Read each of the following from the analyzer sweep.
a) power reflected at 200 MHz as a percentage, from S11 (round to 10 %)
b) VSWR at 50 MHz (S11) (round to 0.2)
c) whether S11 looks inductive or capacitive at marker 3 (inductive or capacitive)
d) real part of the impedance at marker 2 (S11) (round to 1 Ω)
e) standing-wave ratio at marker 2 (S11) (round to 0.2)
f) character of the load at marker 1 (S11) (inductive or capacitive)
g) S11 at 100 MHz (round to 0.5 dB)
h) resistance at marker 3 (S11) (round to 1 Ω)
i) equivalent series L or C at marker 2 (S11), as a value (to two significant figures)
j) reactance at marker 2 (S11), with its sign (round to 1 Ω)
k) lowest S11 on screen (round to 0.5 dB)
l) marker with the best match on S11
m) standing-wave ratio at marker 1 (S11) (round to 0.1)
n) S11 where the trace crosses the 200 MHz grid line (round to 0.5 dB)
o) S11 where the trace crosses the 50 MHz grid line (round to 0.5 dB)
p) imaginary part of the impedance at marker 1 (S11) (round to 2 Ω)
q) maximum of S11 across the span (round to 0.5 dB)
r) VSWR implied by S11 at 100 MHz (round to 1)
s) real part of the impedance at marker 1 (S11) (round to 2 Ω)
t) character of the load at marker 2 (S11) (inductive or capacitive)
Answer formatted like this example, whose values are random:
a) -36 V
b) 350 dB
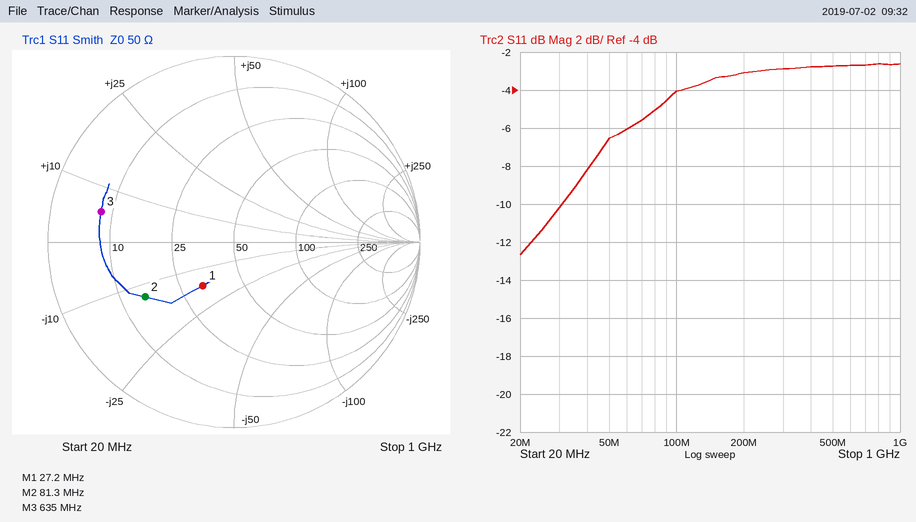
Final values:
a) 50 %
b) 2.8
c) inductive
d) 15 Ω
e) 3.6
f) capacitive
g) -4.0 dB
h) 8 Ω
i) 150 pF
j) -13 Ω
k) -12.5 dB
l) marker 1
m) 1.8
n) -3.0 dB
o) -6.5 dB
p) -16 Ω
q) -2.5 dB
r) 4
s) 32 Ω
t) capacitive
